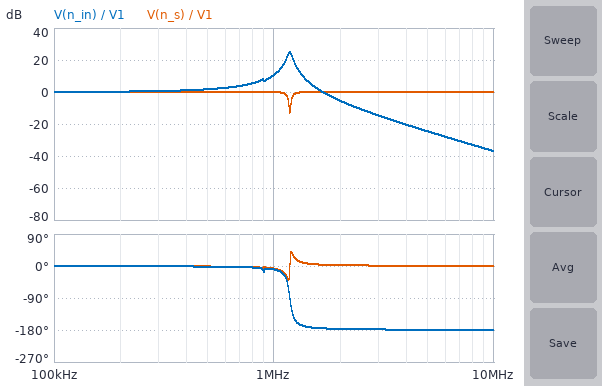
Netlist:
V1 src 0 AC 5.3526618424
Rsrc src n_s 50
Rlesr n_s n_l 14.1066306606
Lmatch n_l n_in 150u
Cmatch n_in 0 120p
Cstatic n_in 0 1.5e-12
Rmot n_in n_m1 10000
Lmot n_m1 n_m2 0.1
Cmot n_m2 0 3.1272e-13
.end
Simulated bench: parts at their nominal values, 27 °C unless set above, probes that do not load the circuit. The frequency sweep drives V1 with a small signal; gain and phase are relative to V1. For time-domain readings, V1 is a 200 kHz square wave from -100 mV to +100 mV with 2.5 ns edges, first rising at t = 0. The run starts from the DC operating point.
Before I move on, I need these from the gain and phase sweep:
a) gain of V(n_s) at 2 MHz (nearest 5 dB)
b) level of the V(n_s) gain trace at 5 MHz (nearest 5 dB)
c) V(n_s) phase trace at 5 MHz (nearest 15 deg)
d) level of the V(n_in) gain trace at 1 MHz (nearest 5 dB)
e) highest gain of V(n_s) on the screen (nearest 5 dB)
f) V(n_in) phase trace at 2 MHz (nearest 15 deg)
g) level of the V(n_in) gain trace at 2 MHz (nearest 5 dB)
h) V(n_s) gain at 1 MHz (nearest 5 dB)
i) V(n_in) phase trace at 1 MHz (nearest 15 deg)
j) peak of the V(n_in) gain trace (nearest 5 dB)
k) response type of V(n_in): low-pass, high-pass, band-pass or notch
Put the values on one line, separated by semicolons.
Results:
0 dB; 0 dB; 0 deg; 10 dB; 0 dB; -180 deg; -5 dB; 0 dB; -15 deg; 25 dB; band-pass
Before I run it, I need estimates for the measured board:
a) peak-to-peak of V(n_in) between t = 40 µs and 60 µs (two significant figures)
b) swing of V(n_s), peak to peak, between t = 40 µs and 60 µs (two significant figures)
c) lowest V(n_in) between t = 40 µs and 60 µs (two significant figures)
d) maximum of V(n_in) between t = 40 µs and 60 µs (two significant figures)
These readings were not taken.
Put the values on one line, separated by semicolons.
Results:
430 mV; 210 mV; -220 mV; 220 mV
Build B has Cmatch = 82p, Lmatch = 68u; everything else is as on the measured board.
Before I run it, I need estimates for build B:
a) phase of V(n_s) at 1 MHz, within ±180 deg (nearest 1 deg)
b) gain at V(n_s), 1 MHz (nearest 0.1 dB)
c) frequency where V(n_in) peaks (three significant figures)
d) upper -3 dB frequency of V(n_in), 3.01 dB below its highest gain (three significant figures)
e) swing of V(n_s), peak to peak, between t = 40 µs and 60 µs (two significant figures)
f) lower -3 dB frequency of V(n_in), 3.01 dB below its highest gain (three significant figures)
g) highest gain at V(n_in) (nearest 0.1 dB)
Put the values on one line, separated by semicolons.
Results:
-2 deg; 0 dB; 2.11 MHz; 2.18 MHz; 220 mV; 2.03 MHz; 23.0 dB
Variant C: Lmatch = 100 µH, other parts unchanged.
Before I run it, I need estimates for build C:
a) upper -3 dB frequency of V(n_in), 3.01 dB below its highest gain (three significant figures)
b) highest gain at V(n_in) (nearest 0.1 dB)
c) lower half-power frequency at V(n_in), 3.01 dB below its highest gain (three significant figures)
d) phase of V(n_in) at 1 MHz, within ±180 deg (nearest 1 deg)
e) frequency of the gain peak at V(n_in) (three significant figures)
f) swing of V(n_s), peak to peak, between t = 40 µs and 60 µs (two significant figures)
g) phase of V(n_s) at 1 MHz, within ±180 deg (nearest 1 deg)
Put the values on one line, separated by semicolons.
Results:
1.49 MHz; 23.0 dB; 1.39 MHz; -5 deg; 1.44 MHz; 230 mV; -4 deg
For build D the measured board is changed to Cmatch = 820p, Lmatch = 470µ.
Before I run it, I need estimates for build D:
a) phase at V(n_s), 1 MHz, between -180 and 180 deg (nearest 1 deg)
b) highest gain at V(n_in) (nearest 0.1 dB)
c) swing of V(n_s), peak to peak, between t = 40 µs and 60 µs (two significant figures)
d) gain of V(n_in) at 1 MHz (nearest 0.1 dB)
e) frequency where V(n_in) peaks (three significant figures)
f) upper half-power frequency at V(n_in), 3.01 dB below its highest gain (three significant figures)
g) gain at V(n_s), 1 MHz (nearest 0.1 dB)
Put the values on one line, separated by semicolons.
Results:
1 deg; 21.4 dB; 230 mV; -23.1 dB; 256 kHz; 266 kHz; 0 dB
